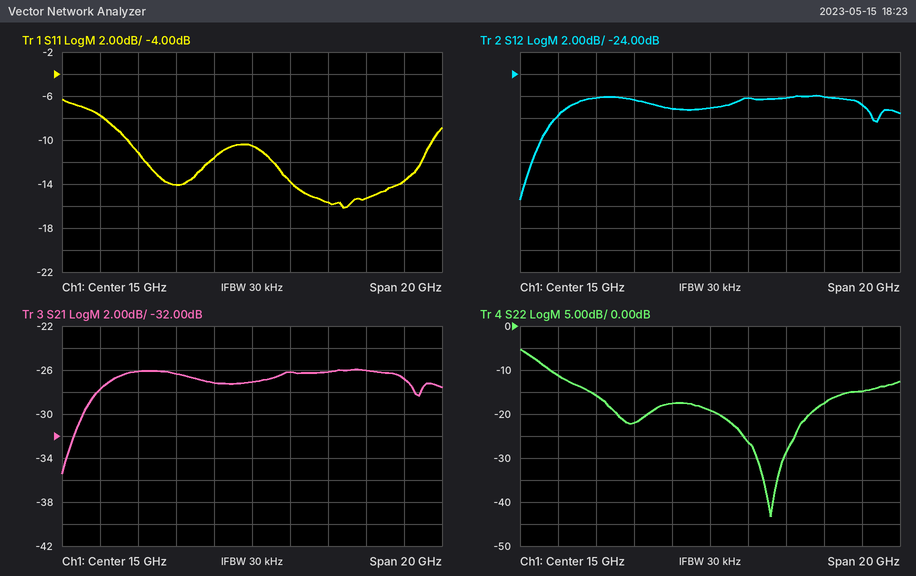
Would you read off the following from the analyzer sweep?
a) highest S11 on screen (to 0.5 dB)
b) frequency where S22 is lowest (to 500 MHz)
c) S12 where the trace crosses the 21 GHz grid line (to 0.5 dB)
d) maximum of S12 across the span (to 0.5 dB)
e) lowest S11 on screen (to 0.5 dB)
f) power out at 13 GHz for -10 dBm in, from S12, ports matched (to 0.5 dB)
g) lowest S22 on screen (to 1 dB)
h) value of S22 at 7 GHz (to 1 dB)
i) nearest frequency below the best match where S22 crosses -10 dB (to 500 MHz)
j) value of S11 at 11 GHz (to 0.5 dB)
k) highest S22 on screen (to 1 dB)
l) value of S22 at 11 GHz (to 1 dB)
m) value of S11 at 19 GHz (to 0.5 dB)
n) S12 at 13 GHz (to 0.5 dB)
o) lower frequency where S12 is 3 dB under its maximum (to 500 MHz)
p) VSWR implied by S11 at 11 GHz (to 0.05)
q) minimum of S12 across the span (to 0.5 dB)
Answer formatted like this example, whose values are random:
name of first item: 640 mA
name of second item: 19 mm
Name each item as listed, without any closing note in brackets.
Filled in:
highest S11 on screen: -6.5 dB
frequency where S22 is lowest: 18.0 GHz
S12 where the trace crosses the 21 GHz grid line: -26.0 dB
maximum of S12 across the span: -26.0 dB
lowest S11 on screen: -16.0 dB
power out at 13 GHz for -10 dBm in, from S12, ports matched: -37.0 dBm
lowest S22 on screen: -43 dB
value of S22 at 7 GHz: -11 dB
nearest frequency below the best match where S22 crosses -10 dB: 6.5 GHz
value of S11 at 11 GHz: -14.0 dB
highest S22 on screen: -5 dB
value of S22 at 11 GHz: -22 dB
value of S11 at 19 GHz: -15.5 dB
S12 at 13 GHz: -27.0 dB
lower frequency where S12 is 3 dB under its maximum: 6.5 GHz
VSWR implied by S11 at 11 GHz: 1.50
minimum of S12 across the span: -35.5 dB
